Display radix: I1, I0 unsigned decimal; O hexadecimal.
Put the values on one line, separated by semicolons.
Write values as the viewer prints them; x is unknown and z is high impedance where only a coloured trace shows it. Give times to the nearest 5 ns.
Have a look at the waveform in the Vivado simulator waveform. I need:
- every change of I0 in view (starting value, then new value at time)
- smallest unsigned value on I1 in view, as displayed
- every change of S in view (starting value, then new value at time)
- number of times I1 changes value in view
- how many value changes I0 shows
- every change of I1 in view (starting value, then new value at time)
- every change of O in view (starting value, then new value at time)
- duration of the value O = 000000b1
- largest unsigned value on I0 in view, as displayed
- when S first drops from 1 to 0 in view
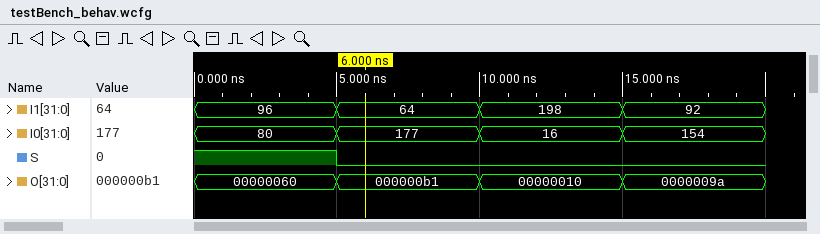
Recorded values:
80, 177 at 5 ns, 16 at 10 ns, 154 at 15 ns; 64; 1, 0 at 5 ns; 3; 3; 96, 64 at 5 ns, 198 at 10 ns, 92 at 15 ns; 00000060, 000000b1 at 5 ns, 00000010 at 10 ns, 0000009a at 15 ns; 5 ns; 177; 5 ns
